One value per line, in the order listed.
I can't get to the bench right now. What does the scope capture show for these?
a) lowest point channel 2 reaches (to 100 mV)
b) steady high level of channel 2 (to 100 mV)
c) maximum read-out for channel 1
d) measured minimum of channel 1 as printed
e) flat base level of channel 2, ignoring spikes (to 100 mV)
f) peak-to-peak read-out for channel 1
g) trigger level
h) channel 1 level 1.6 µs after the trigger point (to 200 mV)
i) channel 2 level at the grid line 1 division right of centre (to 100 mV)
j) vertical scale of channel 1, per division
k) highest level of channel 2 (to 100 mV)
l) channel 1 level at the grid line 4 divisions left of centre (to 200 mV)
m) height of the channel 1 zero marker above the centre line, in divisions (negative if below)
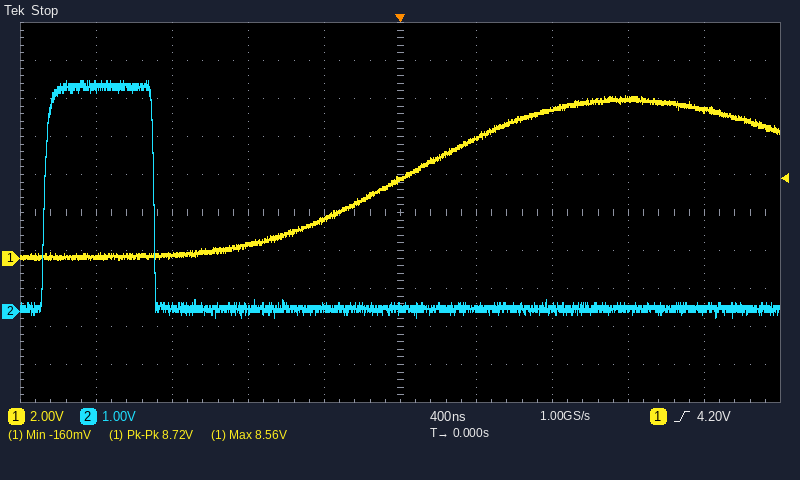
-200 mV
5.9 V
8.56 V
-160 mV
100 mV
8.72 V
4.20 V
7.8 V
100 mV
2 V
6.1 V
200 mV
-1.2 div
